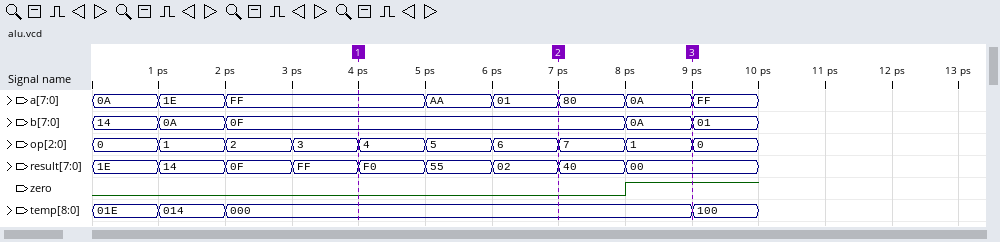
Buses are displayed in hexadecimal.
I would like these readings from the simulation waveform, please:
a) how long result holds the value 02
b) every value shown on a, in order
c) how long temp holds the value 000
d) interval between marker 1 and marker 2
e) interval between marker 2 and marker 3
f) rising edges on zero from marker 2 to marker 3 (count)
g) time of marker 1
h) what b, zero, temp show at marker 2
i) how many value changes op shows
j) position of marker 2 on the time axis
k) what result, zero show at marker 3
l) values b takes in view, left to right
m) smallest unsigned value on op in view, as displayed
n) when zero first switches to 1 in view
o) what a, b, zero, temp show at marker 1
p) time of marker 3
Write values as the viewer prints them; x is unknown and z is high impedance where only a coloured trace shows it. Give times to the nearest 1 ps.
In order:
1 ps
0A, 1E, FF, AA, 01, 80, 0A, FF
7 ps
3 ps
2 ps
1
4 ps
b=0F, zero=0, temp=000
9
7 ps
result=00, zero=1
14, 0A, 0F, 0A, 01
0
8 ps
a=FF, b=0F, zero=0, temp=000
9 ps
